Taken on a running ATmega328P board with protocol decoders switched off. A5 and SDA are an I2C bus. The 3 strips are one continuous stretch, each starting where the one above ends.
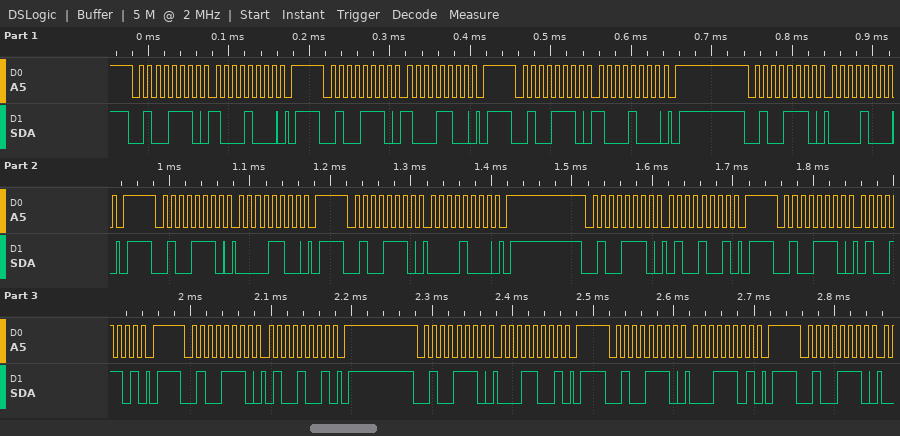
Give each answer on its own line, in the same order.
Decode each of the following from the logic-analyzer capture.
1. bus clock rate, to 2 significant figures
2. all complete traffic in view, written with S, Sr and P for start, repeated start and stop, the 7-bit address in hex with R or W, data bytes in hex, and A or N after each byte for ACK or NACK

100 kHz
S 27W A 88 A P S 27W A 8C A P S 27W A 88 A P S 27W A 08 A P S 27W A 0C A P S 27W A 08 A P S 27W A 49 A P S 27W A 4D A P S 27W A 49 A P S 27W A 19 A P S 27W A 1D A P S 27W A
